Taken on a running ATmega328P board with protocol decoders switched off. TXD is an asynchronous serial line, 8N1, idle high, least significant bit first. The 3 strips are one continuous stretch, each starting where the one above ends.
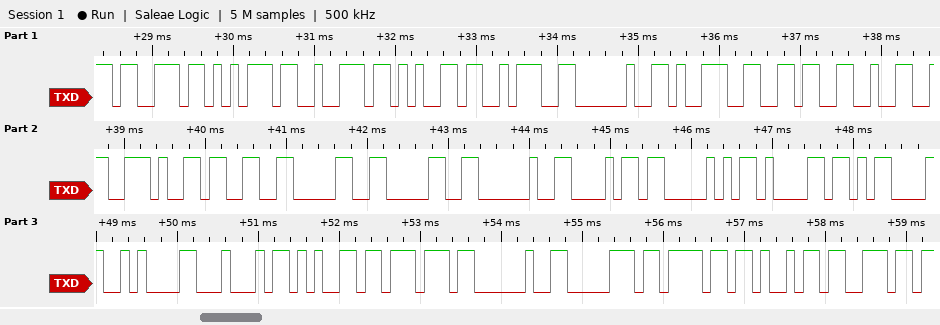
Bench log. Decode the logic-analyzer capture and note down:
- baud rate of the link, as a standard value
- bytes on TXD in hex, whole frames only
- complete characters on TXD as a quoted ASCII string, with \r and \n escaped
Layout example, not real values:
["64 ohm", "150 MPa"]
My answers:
["9600 baud", "73 75 72 65 3A 20 39 36 32 2E 33 30 30 20 68 50 61 0D 0A 44 65 77 20 70 6F 69 6E", "\"sure: 962.300 hPa\\r\\nDew poin\""]
